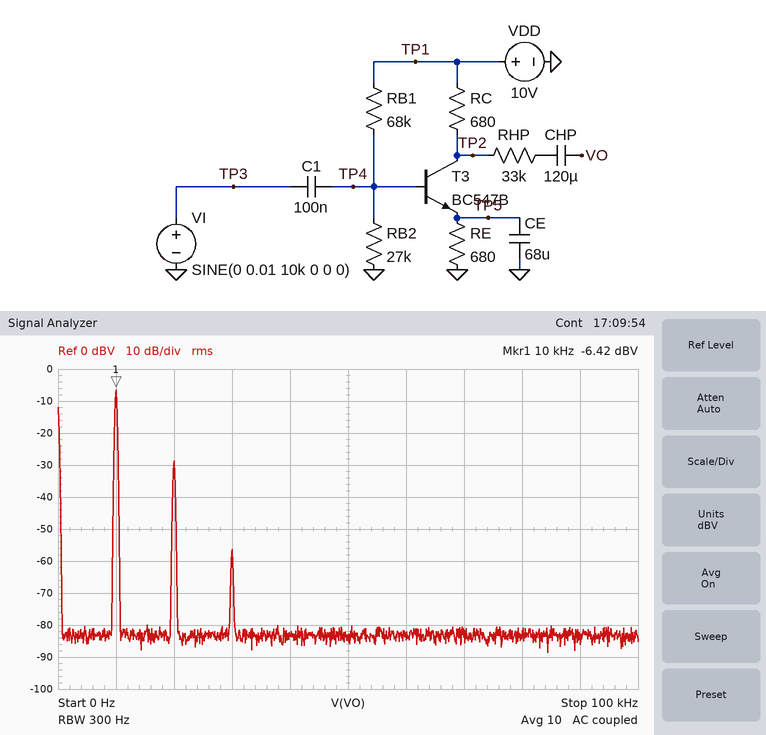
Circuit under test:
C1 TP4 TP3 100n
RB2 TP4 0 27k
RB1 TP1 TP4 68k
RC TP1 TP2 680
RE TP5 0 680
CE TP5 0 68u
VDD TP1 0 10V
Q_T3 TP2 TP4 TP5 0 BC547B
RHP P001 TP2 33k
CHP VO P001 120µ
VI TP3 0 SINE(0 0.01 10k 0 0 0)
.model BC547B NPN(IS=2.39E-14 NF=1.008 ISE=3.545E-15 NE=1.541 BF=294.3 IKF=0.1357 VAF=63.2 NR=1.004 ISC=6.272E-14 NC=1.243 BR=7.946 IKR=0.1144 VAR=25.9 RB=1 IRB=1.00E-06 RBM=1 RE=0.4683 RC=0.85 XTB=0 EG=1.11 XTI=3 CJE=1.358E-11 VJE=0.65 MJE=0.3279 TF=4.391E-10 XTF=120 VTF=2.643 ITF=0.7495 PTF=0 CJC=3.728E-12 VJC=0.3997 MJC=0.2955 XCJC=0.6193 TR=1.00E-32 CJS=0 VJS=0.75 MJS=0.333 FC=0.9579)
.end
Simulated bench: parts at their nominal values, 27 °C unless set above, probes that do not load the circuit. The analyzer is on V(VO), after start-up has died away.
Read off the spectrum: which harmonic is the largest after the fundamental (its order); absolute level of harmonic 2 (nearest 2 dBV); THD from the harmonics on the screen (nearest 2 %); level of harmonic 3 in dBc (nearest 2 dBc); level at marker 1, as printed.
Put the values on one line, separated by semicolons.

2; -28 dBV; 8 %; -50 dBc; -6.42 dBV
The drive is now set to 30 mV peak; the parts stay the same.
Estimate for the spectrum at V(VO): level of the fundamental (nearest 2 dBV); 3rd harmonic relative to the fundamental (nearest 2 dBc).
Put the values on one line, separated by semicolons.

2 dBV; -30 dBc
